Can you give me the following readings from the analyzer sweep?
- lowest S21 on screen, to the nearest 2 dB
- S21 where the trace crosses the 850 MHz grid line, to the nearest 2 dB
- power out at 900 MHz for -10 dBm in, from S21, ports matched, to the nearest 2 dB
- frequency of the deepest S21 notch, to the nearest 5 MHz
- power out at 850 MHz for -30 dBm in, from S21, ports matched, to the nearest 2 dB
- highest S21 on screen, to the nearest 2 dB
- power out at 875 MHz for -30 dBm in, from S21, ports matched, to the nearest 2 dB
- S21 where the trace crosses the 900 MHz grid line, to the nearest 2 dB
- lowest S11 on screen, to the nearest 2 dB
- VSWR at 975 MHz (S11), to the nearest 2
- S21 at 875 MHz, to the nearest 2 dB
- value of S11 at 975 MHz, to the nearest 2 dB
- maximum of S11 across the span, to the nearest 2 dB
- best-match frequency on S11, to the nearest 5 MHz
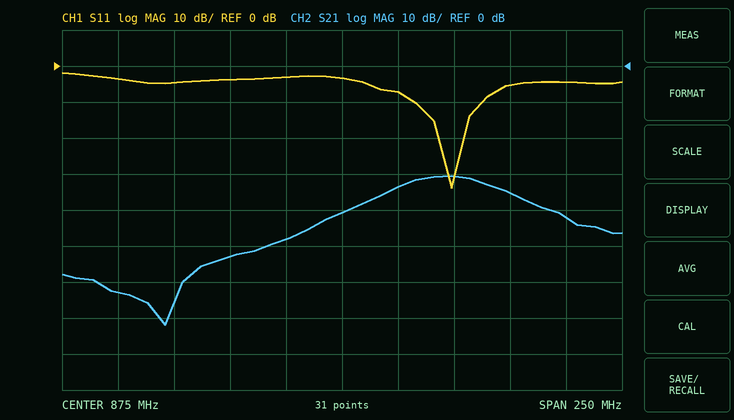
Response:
-72 dB
-48 dB
-44 dBm
795 MHz
-78 dBm
-30 dB
-70 dBm
-34 dB
-34 dB
4
-40 dB
-4 dB
-2 dB
925 MHz
